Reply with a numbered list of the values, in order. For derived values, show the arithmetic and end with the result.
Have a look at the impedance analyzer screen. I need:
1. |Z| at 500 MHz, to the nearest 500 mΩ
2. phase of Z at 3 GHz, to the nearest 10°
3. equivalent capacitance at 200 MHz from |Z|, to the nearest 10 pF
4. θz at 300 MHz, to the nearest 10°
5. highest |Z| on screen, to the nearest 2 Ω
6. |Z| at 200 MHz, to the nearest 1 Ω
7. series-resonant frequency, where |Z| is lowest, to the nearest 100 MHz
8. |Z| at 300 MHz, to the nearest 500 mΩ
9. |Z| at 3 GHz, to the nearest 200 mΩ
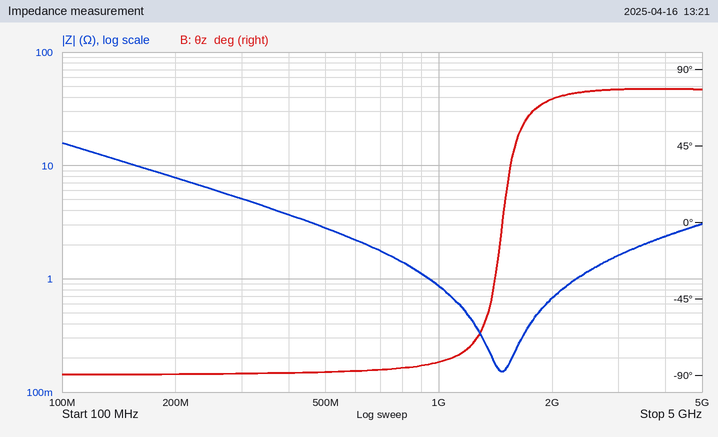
1. 3.0 Ω
2. 80°
3. C = 1/(2π × 200 MHz × 8 Ω) ≈ 100 pF
4. -90°
5. 16 Ω
6. 8 Ω
7. 1.5 GHz
8. 5.0 Ω
9. 1.6 Ω
